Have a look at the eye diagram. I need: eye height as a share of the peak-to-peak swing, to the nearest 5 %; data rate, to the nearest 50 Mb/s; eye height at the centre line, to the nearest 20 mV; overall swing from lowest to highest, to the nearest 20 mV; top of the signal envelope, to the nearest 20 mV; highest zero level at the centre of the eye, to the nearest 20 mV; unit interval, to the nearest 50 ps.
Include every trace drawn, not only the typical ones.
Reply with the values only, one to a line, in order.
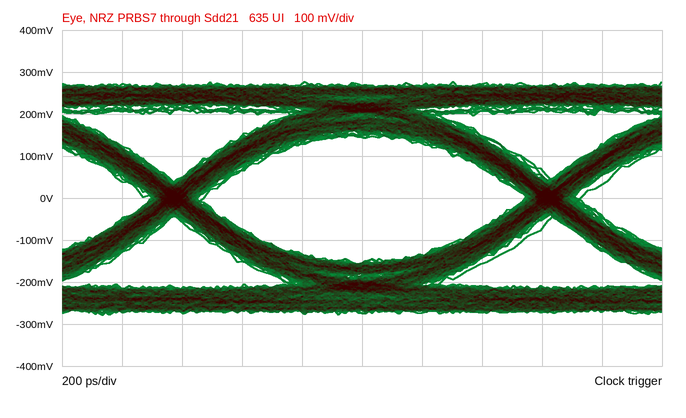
55 %
800 Mb/s
300 mV
560 mV
280 mV
-160 mV
1.25 ns
